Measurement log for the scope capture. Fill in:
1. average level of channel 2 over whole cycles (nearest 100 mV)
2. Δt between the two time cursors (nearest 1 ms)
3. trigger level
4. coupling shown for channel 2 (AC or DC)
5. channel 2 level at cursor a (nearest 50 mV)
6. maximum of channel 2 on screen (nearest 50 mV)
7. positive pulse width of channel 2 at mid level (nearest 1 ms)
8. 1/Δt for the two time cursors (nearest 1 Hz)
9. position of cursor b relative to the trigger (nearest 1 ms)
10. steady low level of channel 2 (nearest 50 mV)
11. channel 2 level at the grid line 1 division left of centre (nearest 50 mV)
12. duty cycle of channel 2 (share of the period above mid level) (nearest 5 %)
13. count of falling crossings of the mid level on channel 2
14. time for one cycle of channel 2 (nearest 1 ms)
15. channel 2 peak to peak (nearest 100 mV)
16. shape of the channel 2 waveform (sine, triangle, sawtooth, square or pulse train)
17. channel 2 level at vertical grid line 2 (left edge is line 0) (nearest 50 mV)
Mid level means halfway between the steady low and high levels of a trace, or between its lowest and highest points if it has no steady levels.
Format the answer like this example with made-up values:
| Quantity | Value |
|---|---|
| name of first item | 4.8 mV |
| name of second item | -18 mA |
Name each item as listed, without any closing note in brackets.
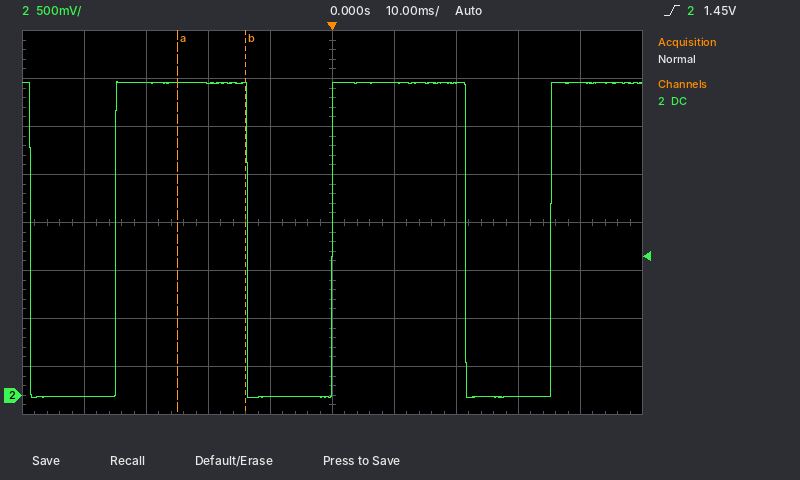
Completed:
| Quantity | Value |
|---|---|
| average level of channel 2 over whole cycles | 2.0 V |
| Δt between the two time cursors | 11 ms |
| trigger level | 1.45 V |
| coupling shown for channel 2 | DC |
| channel 2 level at cursor a | 3.25 V |
| maximum of channel 2 on screen | 3.25 V |
| positive pulse width of channel 2 at mid level | 21 ms |
| 1/Δt for the two time cursors | 91 Hz |
| position of cursor b relative to the trigger | -14 ms |
| steady low level of channel 2 | 0 mV |
| channel 2 level at the grid line 1 division left of centre | 0 mV |
| duty cycle of channel 2 (share of the period above mid level) | 60 % |
| count of falling crossings of the mid level on channel 2 | 3 |
| time for one cycle of channel 2 | 35 ms |
| channel 2 peak to peak | 3.30 V |
| shape of the channel 2 waveform | pulse train |
| channel 2 level at vertical grid line 2 (left edge is line 0) | 3.25 V |
